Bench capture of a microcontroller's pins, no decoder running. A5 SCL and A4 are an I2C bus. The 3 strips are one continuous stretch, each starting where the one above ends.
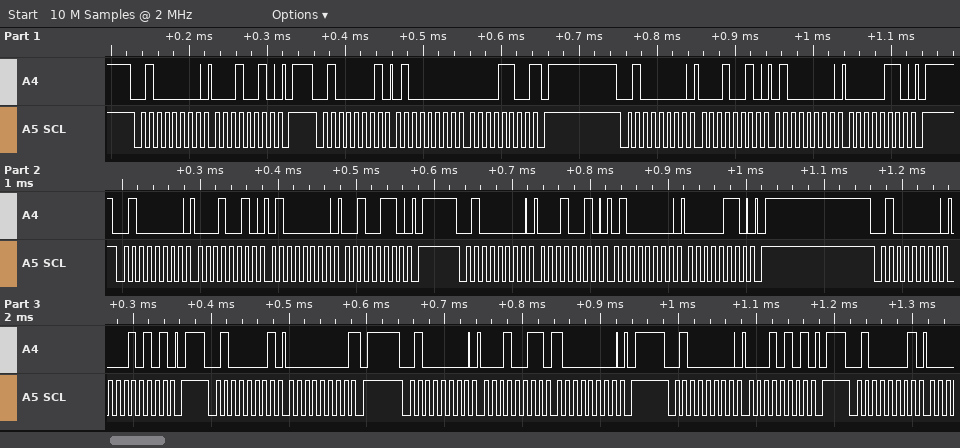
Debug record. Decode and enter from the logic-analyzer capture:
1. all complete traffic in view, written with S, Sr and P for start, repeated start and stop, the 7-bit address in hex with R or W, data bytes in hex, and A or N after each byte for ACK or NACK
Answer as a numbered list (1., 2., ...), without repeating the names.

1. S 20W A 12 A P S 20R A 40 A 0C N P S 20W A 12 A 40 A 06 A P S 20W A 12 A 40 A 26 A P S 20W A 12 A 40 A 06 A P S 20W A 15 A P S 20R A 00 N P S 20W A 13 A 80 A P S 20W A 15 A P S 20R A
